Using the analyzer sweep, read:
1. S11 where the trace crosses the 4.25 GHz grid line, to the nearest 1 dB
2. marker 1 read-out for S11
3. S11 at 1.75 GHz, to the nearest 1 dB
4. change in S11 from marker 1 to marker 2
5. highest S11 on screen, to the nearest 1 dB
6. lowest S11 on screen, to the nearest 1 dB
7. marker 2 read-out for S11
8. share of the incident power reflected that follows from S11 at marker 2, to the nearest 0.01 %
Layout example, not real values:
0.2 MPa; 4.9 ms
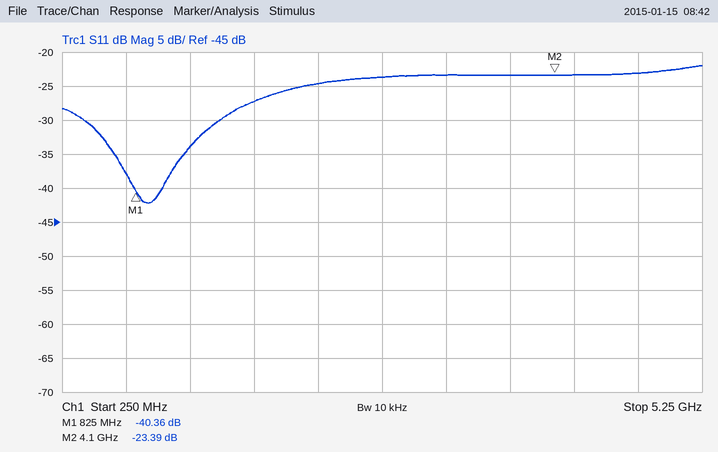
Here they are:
-23 dB; -40.36 dB; -27 dB; 16.97 dB; -22 dB; -42 dB; -23.39 dB; 0.46 %
